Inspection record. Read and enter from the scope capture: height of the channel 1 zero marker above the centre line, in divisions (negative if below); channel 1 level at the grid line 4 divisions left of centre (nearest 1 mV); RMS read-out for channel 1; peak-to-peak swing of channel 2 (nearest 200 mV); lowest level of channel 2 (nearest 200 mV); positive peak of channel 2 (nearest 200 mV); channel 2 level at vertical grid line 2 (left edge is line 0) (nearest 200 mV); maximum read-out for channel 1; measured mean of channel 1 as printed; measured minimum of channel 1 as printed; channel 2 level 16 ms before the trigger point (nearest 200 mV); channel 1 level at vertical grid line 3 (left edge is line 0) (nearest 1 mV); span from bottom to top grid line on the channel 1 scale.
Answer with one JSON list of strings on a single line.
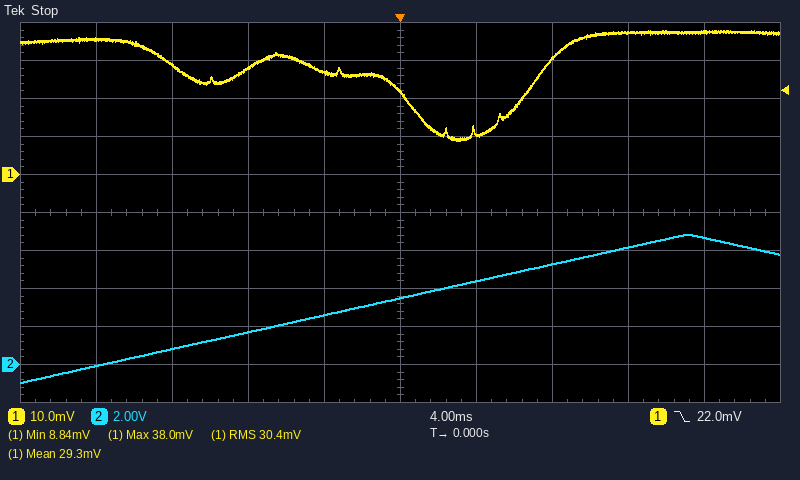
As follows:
["+1.0 div", "36 mV", "30.4 mV", "7.8 V", "-1.0 V", "6.8 V", "800 mV", "38.0 mV", "29.3 mV", "8.84 mV", "0.0 V", "28 mV", "100 mV"]
